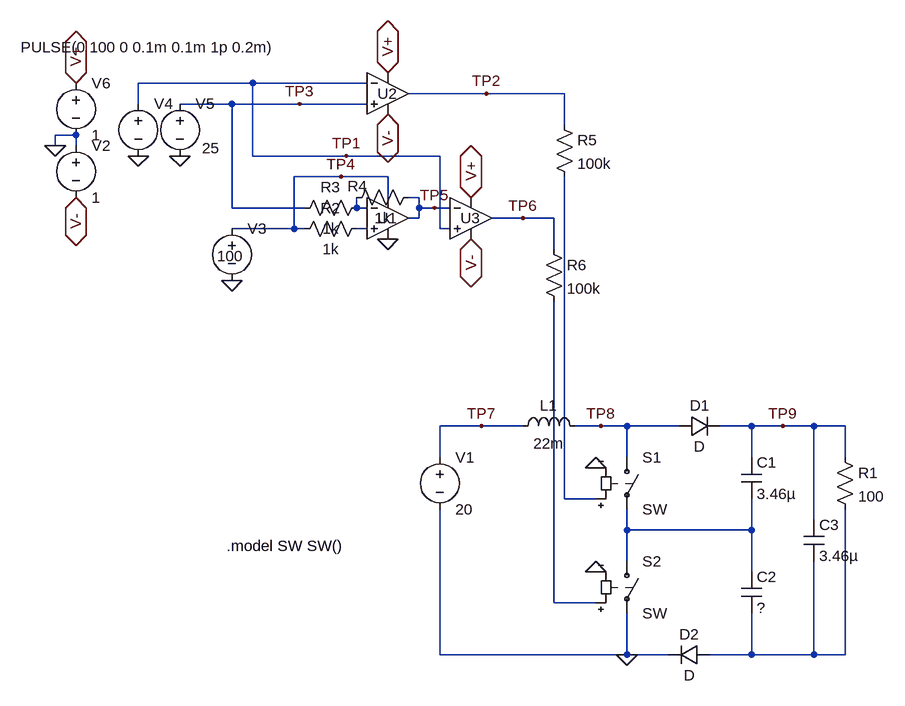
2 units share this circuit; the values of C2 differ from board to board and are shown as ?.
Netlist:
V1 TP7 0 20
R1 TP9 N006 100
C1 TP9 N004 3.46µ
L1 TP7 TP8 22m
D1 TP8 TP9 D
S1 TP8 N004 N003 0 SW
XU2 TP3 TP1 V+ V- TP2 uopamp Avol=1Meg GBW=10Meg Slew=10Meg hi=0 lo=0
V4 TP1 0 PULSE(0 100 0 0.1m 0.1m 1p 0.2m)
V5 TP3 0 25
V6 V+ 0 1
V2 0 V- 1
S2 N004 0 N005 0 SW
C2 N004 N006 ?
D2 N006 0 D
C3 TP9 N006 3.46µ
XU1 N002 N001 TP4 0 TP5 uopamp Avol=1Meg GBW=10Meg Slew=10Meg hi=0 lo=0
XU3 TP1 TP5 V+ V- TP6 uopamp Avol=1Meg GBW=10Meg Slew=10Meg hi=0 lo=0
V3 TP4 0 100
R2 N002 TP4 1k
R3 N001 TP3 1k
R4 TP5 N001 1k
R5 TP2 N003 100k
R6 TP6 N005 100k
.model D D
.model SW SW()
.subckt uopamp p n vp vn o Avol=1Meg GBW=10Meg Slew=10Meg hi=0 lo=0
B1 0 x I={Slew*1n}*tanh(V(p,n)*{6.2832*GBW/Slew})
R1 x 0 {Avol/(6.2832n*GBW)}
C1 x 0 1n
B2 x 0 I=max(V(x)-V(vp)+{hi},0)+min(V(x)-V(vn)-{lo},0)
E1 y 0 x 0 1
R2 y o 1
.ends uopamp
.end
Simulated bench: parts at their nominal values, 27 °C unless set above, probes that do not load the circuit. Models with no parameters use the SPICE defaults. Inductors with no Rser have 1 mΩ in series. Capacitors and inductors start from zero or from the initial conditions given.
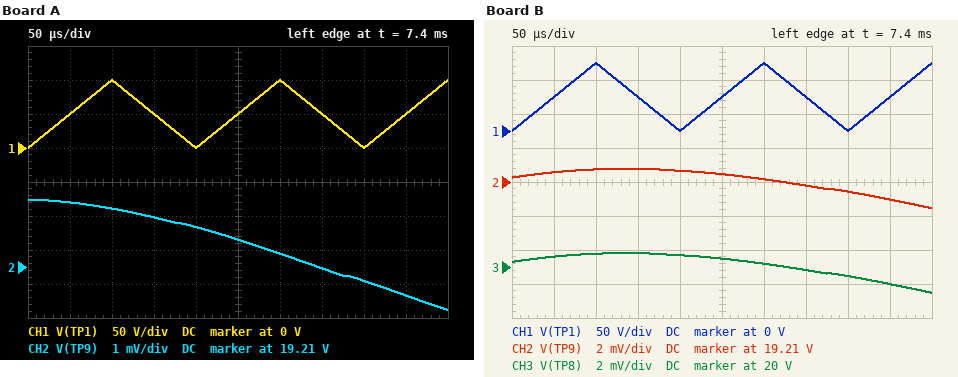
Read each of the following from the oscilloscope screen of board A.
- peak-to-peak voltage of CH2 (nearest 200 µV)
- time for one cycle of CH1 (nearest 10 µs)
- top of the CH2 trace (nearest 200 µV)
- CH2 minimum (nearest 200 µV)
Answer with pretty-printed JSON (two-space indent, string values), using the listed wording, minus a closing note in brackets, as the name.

{
  "peak-to-peak voltage of CH2": "3.2 mV",
  "time for one cycle of CH1": "200 µs",
  "top of the CH2 trace": "19.2140 V",
  "CH2 minimum": "19.2108 V"
}
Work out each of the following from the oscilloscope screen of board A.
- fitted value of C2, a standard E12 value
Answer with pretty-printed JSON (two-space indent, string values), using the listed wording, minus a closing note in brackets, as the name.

{
  "fitted value of C2, a standard E12 value": "1 µF"
}
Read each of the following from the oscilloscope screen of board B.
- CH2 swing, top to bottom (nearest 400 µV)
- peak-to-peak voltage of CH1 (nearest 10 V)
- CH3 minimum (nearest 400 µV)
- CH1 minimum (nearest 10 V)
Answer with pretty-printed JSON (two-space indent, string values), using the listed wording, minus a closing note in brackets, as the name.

{
  "CH2 swing, top to bottom": "2.4 mV",
  "peak-to-peak voltage of CH1": "100 V",
  "CH3 minimum": "20.0024 V",
  "CH1 minimum": "0 V"
}
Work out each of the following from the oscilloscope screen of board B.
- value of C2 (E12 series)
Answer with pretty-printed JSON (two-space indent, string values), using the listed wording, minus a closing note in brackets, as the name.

{
  "value of C2": "1.2 µF"
}
